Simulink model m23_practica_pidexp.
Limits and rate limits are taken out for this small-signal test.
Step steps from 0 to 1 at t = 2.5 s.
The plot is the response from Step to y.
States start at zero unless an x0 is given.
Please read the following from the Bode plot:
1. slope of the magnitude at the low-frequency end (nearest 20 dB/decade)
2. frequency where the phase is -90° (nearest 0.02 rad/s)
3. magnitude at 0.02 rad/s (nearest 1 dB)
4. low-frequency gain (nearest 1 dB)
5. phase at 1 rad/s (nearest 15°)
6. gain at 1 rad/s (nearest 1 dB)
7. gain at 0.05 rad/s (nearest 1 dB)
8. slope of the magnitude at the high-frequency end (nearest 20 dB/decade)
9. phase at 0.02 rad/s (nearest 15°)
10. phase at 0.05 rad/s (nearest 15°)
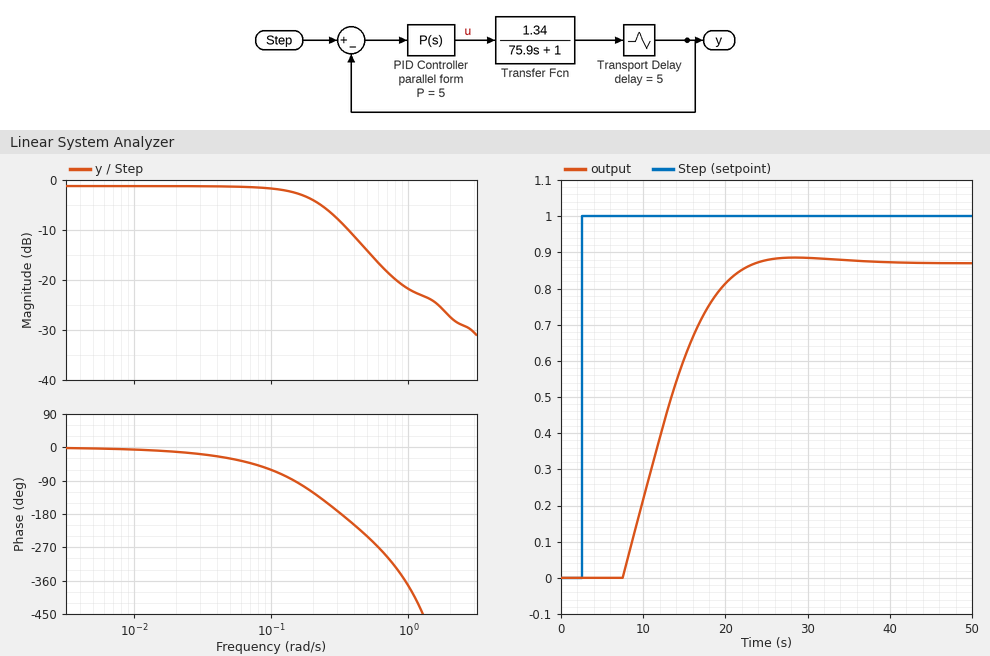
0 dB/decade
0.14 rad/s
-1 dB
-1 dB
-375°
-22 dB
-1 dB
-20 dB/decade
-15°
-30°
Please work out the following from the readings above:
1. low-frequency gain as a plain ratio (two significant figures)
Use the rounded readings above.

0.89
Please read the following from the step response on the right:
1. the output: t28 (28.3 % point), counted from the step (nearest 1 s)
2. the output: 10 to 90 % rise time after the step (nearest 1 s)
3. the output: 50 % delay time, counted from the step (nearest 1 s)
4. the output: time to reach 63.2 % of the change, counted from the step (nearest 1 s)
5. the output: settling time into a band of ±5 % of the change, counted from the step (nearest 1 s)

8 s
10 s
10 s
12 s
18 s
